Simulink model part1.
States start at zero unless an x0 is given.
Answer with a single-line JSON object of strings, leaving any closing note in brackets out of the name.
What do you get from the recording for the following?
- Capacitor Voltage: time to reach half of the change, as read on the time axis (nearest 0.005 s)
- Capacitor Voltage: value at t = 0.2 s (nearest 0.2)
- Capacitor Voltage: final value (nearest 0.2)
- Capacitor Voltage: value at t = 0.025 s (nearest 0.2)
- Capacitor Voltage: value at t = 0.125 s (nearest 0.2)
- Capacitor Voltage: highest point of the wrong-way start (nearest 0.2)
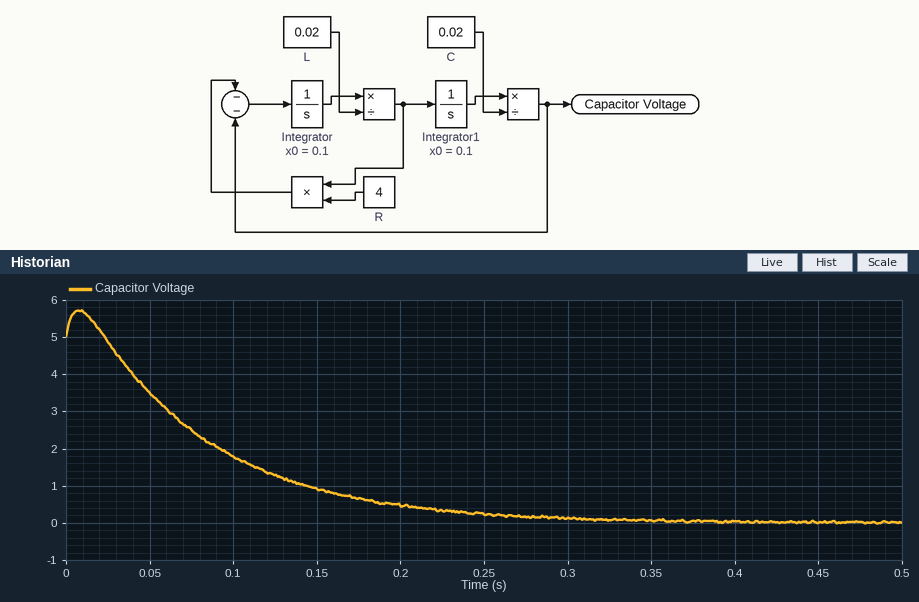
{"Capacitor Voltage: time to reach half of the change, as read on the time axis": "0.075 s", "Capacitor Voltage: value at t = 0.2 s": "0.4", "Capacitor Voltage: final value": "0.0", "Capacitor Voltage: value at t = 0.025 s": "4.8", "Capacitor Voltage: value at t = 0.125 s": "1.2", "Capacitor Voltage: highest point of the wrong-way start": "5.8"}
